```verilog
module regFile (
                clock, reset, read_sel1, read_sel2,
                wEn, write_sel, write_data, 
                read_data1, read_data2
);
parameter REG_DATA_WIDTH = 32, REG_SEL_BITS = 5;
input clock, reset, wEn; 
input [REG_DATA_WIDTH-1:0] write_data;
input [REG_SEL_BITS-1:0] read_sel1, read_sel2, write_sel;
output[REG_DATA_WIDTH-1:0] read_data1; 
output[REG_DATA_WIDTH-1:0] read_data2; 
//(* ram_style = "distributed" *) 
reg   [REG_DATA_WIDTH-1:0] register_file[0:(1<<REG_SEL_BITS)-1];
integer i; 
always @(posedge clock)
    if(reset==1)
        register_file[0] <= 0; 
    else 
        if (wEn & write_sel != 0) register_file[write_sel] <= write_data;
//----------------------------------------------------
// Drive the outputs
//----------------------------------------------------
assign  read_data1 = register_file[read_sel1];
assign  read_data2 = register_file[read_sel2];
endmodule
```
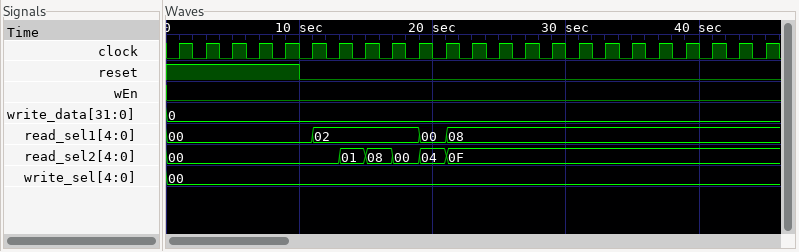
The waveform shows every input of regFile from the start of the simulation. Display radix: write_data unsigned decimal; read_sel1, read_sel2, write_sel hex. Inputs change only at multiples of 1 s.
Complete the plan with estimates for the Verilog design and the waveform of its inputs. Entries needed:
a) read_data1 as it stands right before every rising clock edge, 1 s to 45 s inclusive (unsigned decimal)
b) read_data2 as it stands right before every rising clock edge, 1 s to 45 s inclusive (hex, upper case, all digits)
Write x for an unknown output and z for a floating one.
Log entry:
x, 0, 0, 0, 0, 0, x, x, x, x, 0, x, x, x, x, x, x, x, x, x, x, x, x
x, 00000000, 00000000, 00000000, 00000000, 00000000, 00000000, x, x, 00000000, x, x, x, x, x, x, x, x, x, x, x, x, x
